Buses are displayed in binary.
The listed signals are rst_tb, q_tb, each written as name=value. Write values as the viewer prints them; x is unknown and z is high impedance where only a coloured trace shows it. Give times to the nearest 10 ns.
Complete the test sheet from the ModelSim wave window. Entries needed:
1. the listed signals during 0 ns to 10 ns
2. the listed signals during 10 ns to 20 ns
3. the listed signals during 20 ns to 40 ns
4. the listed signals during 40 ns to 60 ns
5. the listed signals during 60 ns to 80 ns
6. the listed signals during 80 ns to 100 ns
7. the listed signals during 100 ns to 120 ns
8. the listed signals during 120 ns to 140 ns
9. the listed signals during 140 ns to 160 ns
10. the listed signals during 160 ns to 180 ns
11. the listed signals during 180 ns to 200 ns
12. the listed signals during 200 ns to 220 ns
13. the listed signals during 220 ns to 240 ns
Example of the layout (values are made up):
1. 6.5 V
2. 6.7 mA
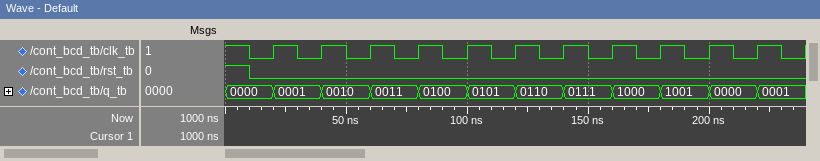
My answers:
1. rst_tb=1, q_tb=0000
2. rst_tb=0, q_tb=0000
3. rst_tb=0, q_tb=0001
4. rst_tb=0, q_tb=0010
5. rst_tb=0, q_tb=0011
6. rst_tb=0, q_tb=0100
7. rst_tb=0, q_tb=0101
8. rst_tb=0, q_tb=0110
9. rst_tb=0, q_tb=0111
10. rst_tb=0, q_tb=1000
11. rst_tb=0, q_tb=1001
12. rst_tb=0, q_tb=0000
13. rst_tb=0, q_tb=0001
